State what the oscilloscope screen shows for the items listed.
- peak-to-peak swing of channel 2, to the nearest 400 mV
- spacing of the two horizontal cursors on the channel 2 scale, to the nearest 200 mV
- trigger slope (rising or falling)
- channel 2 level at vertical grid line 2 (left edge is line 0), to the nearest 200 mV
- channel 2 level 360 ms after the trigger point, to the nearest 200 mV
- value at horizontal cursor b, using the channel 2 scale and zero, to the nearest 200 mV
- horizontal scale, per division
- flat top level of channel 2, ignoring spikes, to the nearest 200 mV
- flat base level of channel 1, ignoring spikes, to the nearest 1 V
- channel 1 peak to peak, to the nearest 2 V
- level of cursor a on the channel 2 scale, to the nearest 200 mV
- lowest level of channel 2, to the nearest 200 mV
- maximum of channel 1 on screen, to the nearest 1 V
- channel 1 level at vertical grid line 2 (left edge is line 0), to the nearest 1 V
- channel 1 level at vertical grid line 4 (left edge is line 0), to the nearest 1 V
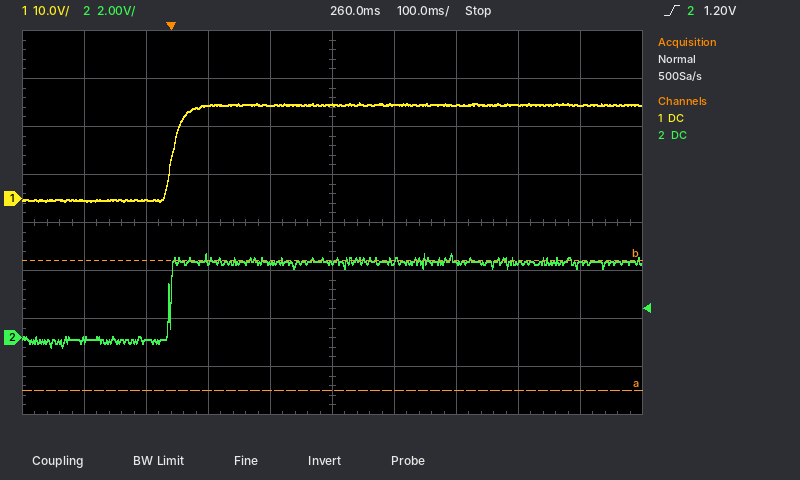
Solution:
4.0 V
5.4 V
rising
-200 mV
3.2 V
3.2 V
100 ms
3.2 V
0 V
20 V
-2.2 V
-400 mV
20 V
0 V
19 V
